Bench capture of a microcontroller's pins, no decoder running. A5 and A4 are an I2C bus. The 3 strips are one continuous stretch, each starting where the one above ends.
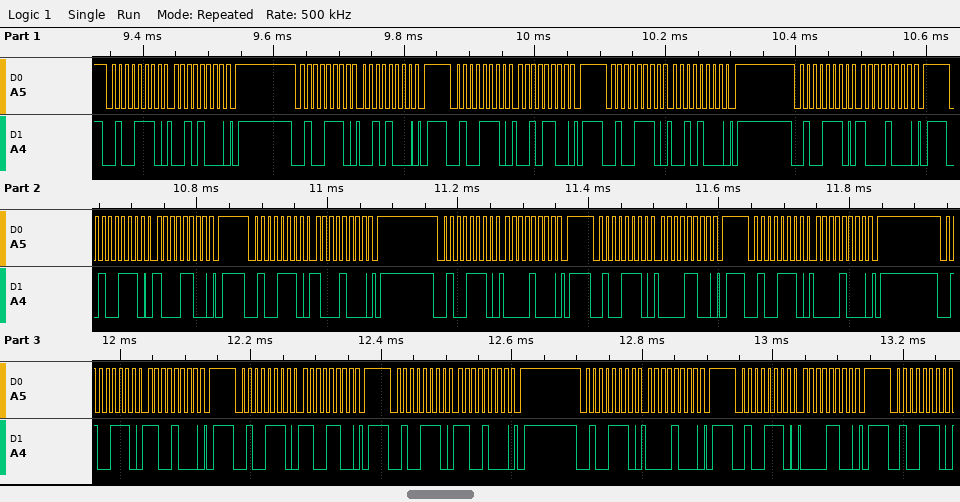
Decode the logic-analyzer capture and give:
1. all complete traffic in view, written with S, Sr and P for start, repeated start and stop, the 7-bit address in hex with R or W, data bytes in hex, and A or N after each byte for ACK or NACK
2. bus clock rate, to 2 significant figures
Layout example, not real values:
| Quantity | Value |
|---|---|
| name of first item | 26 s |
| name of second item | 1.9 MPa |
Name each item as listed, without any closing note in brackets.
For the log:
| Quantity | Value |
|---|---|
| all complete traffic in view, written with S, Sr and P for start, repeated start and stop, the 7-bit address in hex with R or W, data bytes in hex, and A or N after each byte for ACK or NACK | S 27W A 28 A P S 27W A 28 A P S 27W A 2C A P S 27W A 28 A P S 27W A 88 A P S 27W A 8C A P S 27W A 88 A P S 27W A 08 A P S 27W A 0C A P S 27W A 08 A P S 27W A C8 A P S 27W A CC A P S 27W A C8 A P S 27W A 08 A P S 27W A 0C A P S 27W A |
| bus clock rate, to 2 significant figures | 100 kHz |
